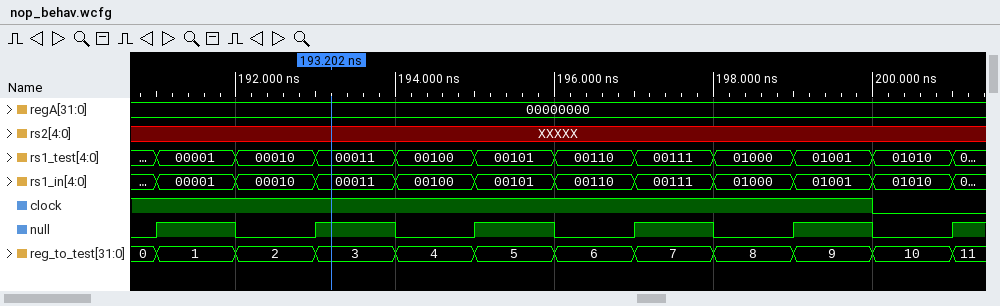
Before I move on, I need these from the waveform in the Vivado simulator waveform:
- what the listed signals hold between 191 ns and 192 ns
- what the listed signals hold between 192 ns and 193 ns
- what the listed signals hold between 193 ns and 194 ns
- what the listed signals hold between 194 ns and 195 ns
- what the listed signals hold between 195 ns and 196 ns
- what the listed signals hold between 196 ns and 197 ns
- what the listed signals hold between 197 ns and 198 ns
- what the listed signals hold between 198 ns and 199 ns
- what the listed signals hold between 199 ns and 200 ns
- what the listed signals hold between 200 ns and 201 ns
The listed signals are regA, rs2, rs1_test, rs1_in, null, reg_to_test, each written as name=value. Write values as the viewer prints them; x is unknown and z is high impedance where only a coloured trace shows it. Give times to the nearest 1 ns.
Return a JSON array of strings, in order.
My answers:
["regA=00000000, rs2=XXXXX, rs1_test=00001, rs1_in=00001, null=1, reg_to_test=1", "regA=00000000, rs2=XXXXX, rs1_test=00010, rs1_in=00010, null=0, reg_to_test=2", "regA=00000000, rs2=XXXXX, rs1_test=00011, rs1_in=00011, null=1, reg_to_test=3", "regA=00000000, rs2=XXXXX, rs1_test=00100, rs1_in=00100, null=0, reg_to_test=4", "regA=00000000, rs2=XXXXX, rs1_test=00101, rs1_in=00101, null=1, reg_to_test=5", "regA=00000000, rs2=XXXXX, rs1_test=00110, rs1_in=00110, null=0, reg_to_test=6", "regA=00000000, rs2=XXXXX, rs1_test=00111, rs1_in=00111, null=1, reg_to_test=7", "regA=00000000, rs2=XXXXX, rs1_test=01000, rs1_in=01000, null=0, reg_to_test=8", "regA=00000000, rs2=XXXXX, rs1_test=01001, rs1_in=01001, null=1, reg_to_test=9", "regA=00000000, rs2=XXXXX, rs1_test=01010, rs1_in=01010, null=0, reg_to_test=10"]
